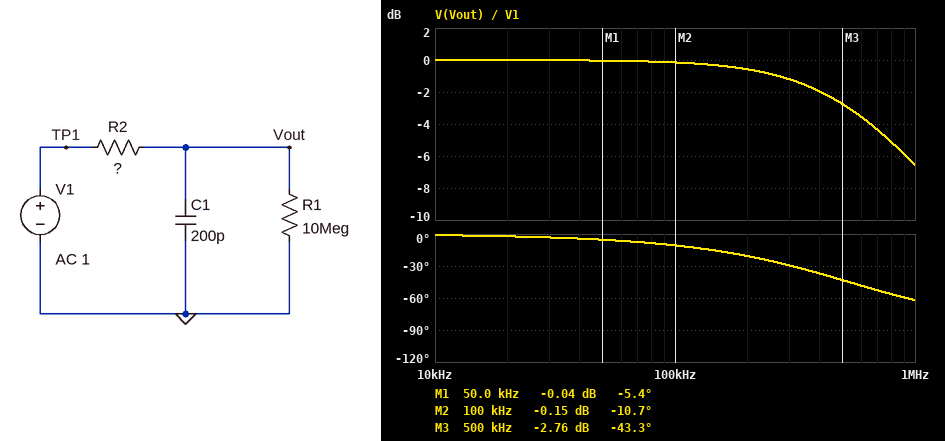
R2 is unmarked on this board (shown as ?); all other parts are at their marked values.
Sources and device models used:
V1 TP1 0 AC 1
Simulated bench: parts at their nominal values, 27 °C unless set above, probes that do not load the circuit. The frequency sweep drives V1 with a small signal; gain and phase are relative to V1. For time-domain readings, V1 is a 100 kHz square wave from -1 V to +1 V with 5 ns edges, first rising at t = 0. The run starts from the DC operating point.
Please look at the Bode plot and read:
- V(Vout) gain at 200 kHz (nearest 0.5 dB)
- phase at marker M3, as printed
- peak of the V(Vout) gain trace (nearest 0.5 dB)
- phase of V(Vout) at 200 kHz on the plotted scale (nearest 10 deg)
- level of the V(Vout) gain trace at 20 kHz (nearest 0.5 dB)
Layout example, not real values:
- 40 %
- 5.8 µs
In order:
- -0.5 dB
- -43.3 deg
- 0 dB
- -20 deg
- 0 dB
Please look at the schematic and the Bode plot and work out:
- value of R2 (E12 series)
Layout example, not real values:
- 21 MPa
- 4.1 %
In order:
- 1.5 kΩ
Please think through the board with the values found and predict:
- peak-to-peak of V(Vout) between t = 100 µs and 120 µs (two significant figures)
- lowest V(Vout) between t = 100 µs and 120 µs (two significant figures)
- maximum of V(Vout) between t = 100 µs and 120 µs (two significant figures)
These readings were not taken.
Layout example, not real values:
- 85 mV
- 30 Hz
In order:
- 2.0 V
- -1.0 V
- 1.0 V
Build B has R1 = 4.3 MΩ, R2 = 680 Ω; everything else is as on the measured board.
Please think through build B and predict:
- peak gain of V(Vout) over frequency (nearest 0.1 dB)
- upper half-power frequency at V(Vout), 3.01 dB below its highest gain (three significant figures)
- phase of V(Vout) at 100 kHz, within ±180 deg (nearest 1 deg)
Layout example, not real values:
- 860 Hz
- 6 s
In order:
- 0 dB
- 1.17 MHz
- -5 deg
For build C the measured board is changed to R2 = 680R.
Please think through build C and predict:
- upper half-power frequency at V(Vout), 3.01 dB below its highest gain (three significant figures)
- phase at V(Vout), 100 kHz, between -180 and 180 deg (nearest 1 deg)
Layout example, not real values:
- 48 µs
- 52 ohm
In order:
- 1.17 MHz
- -5 deg
